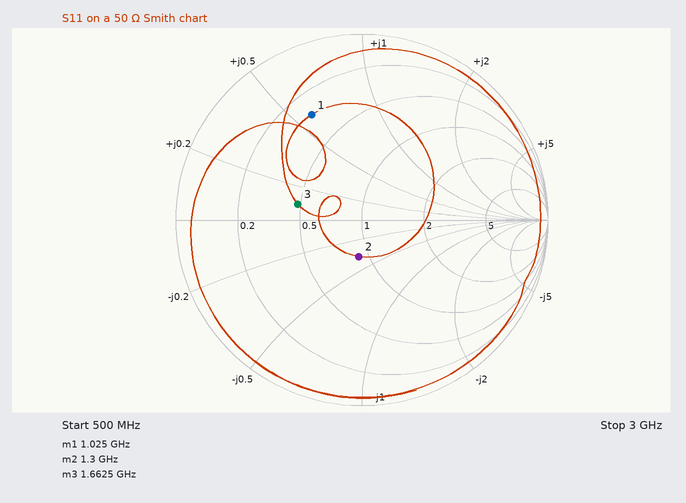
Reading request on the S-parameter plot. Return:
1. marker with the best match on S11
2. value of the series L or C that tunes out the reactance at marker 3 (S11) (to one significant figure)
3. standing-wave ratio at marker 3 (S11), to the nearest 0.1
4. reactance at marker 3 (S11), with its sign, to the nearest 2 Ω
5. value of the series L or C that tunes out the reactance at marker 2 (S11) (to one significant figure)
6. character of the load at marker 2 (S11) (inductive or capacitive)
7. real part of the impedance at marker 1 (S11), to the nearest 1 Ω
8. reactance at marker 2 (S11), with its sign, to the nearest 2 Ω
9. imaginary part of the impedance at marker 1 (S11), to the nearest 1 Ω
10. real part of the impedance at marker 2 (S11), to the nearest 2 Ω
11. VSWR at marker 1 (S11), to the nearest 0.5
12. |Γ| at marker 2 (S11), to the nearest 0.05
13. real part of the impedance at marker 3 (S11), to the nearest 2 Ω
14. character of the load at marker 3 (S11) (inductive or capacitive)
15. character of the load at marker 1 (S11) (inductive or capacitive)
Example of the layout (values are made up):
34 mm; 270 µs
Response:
marker 2; 20 pF; 2.1; +4 Ω; 2 nH; capacitive; 16 Ω; -18 Ω; +29 Ω; 44 Ω; 4.5; 0.20; 24 Ω; inductive; inductive
